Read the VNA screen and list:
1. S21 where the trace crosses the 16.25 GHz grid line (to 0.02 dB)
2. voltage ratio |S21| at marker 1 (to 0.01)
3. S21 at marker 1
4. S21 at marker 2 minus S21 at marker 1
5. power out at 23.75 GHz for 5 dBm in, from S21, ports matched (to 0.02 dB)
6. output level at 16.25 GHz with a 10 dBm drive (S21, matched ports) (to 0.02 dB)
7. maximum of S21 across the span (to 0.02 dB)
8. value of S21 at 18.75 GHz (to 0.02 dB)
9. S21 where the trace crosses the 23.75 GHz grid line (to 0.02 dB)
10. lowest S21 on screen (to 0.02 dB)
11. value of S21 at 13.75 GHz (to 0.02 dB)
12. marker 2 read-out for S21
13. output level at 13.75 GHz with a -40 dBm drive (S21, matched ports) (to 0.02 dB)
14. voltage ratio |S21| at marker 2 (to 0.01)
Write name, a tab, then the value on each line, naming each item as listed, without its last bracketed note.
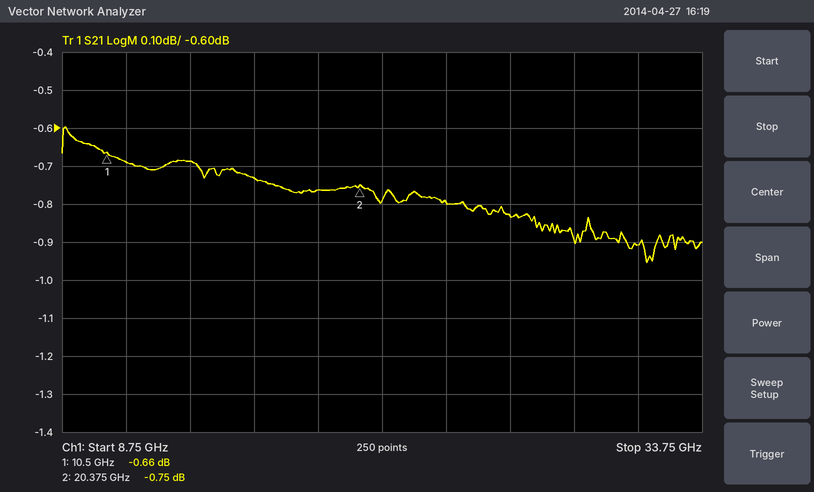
S21 where the trace crosses the 16.25 GHz grid line	-0.74 dB
voltage ratio |S21| at marker 1	0.93
S21 at marker 1	-0.66 dB
S21 at marker 2 minus S21 at marker 1	-0.09 dB
power out at 23.75 GHz for 5 dBm in, from S21, ports matched	4.20 dBm
output level at 16.25 GHz with a 10 dBm drive (S21, matched ports)	9.26 dBm
maximum of S21 across the span	-0.60 dB
value of S21 at 18.75 GHz	-0.76 dB
S21 where the trace crosses the 23.75 GHz grid line	-0.80 dB
lowest S21 on screen	-0.96 dB
value of S21 at 13.75 GHz	-0.68 dB
marker 2 read-out for S21	-0.75 dB
output level at 13.75 GHz with a -40 dBm drive (S21, matched ports)	-40.68 dBm
voltage ratio |S21| at marker 2	0.92
